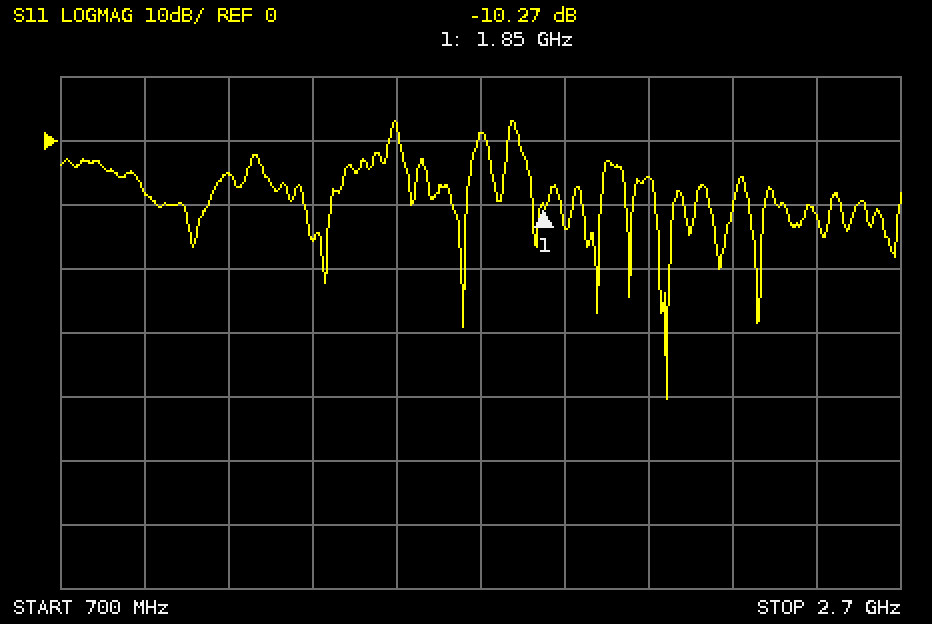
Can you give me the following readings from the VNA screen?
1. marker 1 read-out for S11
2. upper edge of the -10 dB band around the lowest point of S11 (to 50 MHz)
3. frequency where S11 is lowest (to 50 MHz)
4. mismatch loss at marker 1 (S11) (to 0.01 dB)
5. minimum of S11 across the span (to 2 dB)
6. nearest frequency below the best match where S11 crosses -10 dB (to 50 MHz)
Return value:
-10.27 dB
2.15 GHz
2.15 GHz
0.43 dB
-40 dB
2.10 GHz
